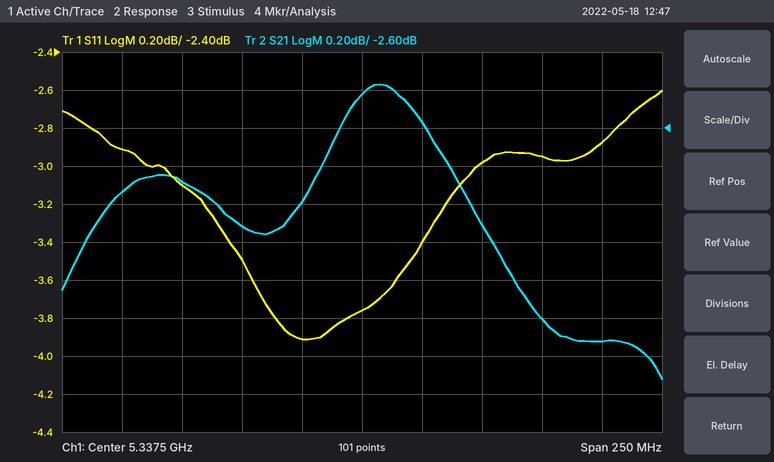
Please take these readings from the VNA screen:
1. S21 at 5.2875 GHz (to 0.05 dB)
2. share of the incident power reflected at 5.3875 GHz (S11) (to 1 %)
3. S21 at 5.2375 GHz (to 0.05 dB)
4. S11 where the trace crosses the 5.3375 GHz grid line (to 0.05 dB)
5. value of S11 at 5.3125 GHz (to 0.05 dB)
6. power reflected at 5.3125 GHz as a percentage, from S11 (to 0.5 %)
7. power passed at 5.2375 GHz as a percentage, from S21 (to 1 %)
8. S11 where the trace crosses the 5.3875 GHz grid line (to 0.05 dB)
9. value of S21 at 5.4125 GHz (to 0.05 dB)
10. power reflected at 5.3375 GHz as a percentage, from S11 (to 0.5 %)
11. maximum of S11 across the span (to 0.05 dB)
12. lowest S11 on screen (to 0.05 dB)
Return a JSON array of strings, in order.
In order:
["-3.10 dB", "50 %", "-2.95 dB", "-3.75 dB", "-3.90 dB", "40.5 %", "51 %", "-3.00 dB", "-3.60 dB", "42.0 %", "-2.60 dB", "-3.90 dB"]
